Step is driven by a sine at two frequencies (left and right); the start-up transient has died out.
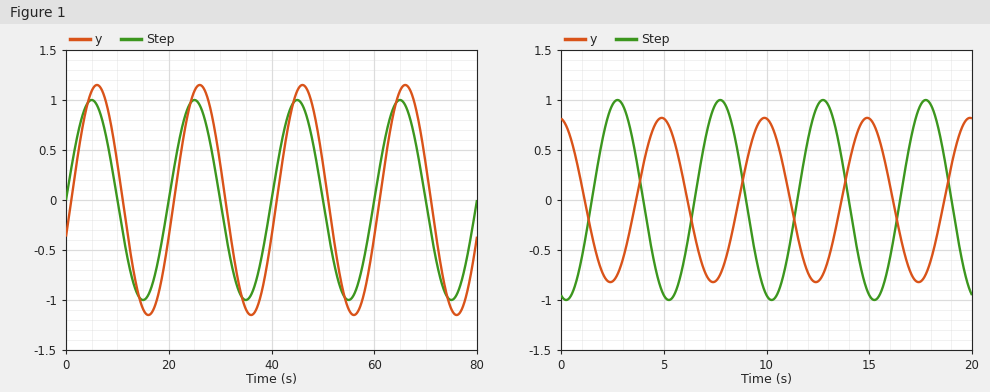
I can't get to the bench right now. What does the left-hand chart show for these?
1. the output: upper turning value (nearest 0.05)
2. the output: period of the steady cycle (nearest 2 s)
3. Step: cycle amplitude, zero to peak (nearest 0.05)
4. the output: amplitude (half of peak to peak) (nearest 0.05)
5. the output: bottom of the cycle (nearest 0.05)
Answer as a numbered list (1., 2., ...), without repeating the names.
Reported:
1. 1.15
2. 20 s
3. 1.00
4. 1.15
5. -1.15
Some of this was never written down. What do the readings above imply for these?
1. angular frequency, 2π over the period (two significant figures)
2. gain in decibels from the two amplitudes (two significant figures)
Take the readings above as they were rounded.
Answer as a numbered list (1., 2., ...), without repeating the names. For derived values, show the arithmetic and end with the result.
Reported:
1. 2π / 20 = 0.31 rad/s
2. 20 log10(1.15 / 1) = 1.2 dB
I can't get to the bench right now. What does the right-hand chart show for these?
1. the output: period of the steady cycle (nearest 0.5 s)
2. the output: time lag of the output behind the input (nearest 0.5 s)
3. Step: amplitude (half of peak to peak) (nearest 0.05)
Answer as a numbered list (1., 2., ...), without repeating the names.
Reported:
1. 5.0 s
2. 2.0 s
3. 1.00
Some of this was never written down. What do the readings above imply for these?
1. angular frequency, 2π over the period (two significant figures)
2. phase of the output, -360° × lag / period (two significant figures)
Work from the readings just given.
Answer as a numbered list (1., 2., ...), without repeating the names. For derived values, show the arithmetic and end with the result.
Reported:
1. 2π / 5 = 1.3 rad/s
2. -360 × 2 / 5 = -140°
